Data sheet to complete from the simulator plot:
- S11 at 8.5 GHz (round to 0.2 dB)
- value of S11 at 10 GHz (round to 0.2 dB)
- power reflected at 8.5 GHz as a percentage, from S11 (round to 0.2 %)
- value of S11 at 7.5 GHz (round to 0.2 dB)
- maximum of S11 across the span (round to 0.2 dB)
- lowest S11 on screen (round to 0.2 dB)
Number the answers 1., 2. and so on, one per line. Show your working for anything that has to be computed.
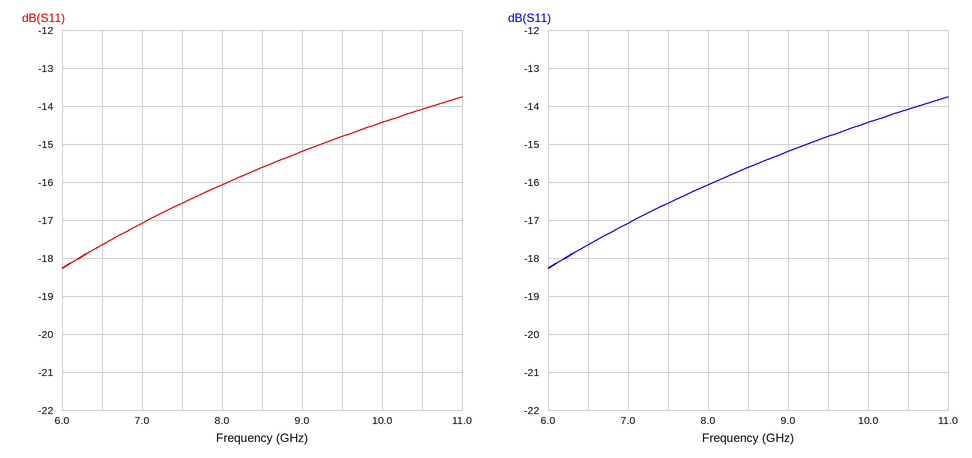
1. -15.6 dB
2. -14.4 dB
3. 10^(-15.6/10) ≈ 2.8 %
4. -16.6 dB
5. -13.8 dB
6. -18.2 dB
